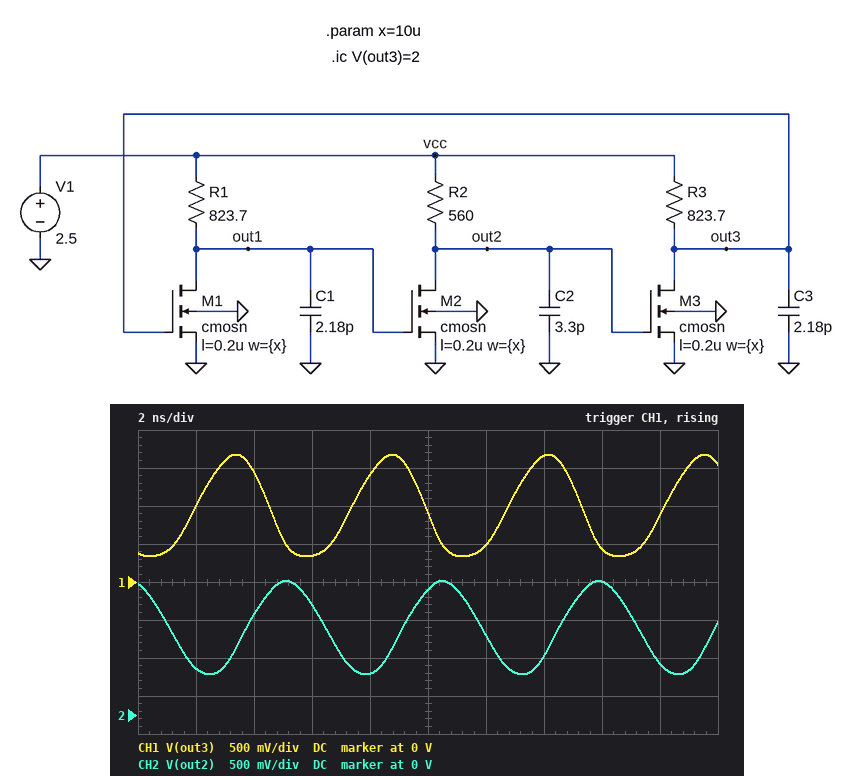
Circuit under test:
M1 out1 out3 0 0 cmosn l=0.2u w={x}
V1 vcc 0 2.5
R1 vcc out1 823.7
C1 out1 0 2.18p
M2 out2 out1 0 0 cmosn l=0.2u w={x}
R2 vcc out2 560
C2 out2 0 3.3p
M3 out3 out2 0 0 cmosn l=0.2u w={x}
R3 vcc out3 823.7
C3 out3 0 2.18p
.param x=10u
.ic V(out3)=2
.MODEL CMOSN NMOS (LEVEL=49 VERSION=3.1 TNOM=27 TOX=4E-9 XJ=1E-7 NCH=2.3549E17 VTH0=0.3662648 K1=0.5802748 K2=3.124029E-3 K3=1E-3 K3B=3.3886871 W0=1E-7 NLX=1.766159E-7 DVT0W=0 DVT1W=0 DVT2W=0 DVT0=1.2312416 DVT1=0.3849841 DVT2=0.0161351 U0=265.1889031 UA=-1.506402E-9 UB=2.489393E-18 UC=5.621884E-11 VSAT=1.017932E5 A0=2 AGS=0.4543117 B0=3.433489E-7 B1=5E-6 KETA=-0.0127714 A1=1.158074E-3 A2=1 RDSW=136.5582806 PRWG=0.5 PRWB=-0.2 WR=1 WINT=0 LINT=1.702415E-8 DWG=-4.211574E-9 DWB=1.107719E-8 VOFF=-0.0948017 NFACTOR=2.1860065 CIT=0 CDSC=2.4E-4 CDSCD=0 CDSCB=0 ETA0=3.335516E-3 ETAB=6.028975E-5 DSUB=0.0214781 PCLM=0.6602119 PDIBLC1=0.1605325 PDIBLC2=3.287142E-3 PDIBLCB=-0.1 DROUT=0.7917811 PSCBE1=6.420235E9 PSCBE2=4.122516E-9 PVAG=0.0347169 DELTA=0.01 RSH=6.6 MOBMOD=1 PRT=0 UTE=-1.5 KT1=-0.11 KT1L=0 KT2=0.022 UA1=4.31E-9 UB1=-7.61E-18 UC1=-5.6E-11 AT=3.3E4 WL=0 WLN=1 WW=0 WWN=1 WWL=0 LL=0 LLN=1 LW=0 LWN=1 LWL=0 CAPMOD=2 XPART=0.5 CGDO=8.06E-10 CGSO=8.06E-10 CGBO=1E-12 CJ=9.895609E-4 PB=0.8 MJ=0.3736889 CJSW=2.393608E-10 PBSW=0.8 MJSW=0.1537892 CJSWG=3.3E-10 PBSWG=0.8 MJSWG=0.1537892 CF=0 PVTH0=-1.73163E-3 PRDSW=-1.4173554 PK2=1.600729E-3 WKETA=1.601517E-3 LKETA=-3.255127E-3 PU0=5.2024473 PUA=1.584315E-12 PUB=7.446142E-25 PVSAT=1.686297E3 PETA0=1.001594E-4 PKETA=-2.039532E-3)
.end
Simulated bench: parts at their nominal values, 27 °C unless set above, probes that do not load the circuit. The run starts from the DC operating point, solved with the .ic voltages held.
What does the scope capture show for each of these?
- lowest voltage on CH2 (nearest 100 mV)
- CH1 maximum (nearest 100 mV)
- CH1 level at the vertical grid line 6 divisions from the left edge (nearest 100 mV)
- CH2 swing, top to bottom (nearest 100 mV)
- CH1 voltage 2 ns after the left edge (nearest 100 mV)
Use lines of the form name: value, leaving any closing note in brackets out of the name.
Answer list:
lowest voltage on CH2: 500 mV
CH1 maximum: 1.7 V
CH1 level at the vertical grid line 6 divisions from the left edge: 500 mV
CH2 swing, top to bottom: 1.2 V
CH1 voltage 2 ns after the left edge: 1.0 V
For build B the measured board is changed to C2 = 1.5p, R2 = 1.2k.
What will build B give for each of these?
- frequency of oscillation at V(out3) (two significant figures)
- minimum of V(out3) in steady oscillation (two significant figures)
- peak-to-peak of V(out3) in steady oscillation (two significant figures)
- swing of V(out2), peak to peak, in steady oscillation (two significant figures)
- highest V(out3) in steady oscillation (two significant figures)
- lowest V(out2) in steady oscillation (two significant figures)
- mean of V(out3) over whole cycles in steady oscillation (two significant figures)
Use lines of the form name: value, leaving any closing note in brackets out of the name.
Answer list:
frequency of oscillation at V(out3): 210 MHz
minimum of V(out3) in steady oscillation: 380 mV
peak-to-peak of V(out3) in steady oscillation: 1.4 V
swing of V(out2), peak to peak, in steady oscillation: 1.5 V
highest V(out3) in steady oscillation: 1.8 V
lowest V(out2) in steady oscillation: 230 mV
mean of V(out3) over whole cycles in steady oscillation: 1.1 V
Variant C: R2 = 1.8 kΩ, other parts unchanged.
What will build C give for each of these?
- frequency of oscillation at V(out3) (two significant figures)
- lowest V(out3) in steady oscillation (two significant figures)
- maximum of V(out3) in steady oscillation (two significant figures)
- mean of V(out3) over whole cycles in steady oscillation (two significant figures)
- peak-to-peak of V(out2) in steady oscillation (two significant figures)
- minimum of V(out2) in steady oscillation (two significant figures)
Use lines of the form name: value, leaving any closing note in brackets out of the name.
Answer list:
frequency of oscillation at V(out3): 140 MHz
lowest V(out3) in steady oscillation: 600 mV
maximum of V(out3) in steady oscillation: 2.0 V
mean of V(out3) over whole cycles in steady oscillation: 1.4 V
peak-to-peak of V(out2) in steady oscillation: 1.1 V
minimum of V(out2) in steady oscillation: 290 mV
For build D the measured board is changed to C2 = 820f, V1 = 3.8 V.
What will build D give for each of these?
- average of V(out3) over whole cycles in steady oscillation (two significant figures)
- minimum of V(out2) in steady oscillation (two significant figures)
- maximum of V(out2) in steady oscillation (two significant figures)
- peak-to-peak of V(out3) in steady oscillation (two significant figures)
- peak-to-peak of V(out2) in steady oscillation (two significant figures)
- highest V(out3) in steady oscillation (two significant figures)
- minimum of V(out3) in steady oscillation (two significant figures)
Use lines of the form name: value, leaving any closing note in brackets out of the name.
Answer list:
average of V(out3) over whole cycles in steady oscillation: 1.2 V
minimum of V(out2) in steady oscillation: 710 mV
maximum of V(out2) in steady oscillation: 2.4 V
peak-to-peak of V(out3) in steady oscillation: 1.4 V
peak-to-peak of V(out2) in steady oscillation: 1.7 V
highest V(out3) in steady oscillation: 1.9 V
minimum of V(out3) in steady oscillation: 550 mV
